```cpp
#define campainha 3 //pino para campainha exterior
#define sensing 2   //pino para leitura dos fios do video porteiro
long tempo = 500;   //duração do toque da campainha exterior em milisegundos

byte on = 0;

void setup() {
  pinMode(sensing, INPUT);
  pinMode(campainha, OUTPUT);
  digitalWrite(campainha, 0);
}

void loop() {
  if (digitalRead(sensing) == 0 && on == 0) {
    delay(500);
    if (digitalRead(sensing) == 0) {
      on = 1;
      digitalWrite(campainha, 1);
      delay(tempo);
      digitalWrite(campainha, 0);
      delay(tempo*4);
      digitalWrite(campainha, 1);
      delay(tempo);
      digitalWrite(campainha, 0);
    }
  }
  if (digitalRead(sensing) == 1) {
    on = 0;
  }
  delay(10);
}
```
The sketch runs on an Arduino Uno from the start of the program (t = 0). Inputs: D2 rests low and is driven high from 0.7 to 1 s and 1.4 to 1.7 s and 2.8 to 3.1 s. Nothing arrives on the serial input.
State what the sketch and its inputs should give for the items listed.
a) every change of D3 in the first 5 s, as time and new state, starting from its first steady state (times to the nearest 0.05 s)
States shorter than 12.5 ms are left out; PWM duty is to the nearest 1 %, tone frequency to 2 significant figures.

0 s low; 0.5 s high; 1 s low; 3 s high; 3.5 s low
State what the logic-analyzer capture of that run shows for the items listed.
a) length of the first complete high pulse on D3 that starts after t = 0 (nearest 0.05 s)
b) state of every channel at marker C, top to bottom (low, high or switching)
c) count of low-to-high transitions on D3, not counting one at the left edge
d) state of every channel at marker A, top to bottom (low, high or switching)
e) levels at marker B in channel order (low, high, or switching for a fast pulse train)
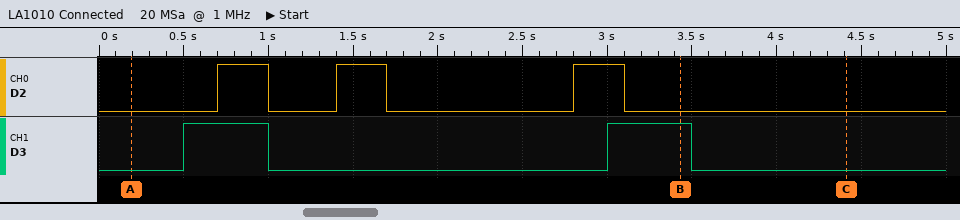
0.50 s
D2 low, D3 low
2
D2 low, D3 low
D2 low, D3 high
